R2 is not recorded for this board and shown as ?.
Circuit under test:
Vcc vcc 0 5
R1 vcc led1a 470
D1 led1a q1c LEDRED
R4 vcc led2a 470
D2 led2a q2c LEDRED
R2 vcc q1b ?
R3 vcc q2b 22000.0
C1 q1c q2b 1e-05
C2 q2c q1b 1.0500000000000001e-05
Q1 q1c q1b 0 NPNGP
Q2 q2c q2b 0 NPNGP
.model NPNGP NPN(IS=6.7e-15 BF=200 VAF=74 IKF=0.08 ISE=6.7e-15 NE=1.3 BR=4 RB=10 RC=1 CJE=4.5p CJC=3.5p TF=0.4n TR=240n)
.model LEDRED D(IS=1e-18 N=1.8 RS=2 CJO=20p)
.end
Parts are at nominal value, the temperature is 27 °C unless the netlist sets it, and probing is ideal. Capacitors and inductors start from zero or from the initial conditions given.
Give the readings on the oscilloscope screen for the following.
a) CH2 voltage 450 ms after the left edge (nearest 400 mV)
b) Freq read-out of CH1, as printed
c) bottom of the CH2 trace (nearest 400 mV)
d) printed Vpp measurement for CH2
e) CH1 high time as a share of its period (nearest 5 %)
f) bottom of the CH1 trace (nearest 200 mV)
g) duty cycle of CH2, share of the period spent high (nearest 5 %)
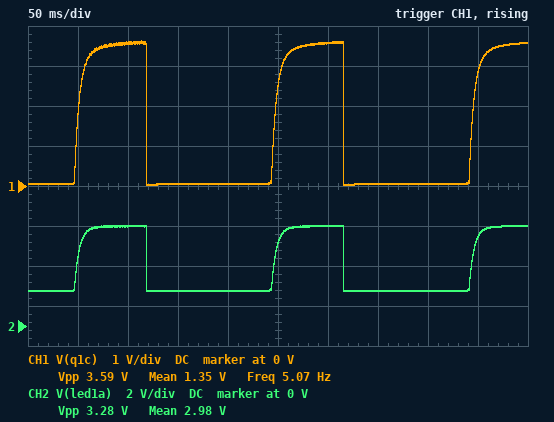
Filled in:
4.4 V
5.07 Hz
1.6 V
3.28 V
35 %
0 V
35 %
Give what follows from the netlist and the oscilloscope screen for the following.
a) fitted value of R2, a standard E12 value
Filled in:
12 kΩ
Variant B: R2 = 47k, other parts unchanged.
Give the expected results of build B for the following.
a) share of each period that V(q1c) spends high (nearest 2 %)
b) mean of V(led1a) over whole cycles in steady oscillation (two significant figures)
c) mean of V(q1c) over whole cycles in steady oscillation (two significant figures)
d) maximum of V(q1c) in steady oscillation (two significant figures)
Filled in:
68 %
4.0 V
2.5 V
3.7 V
